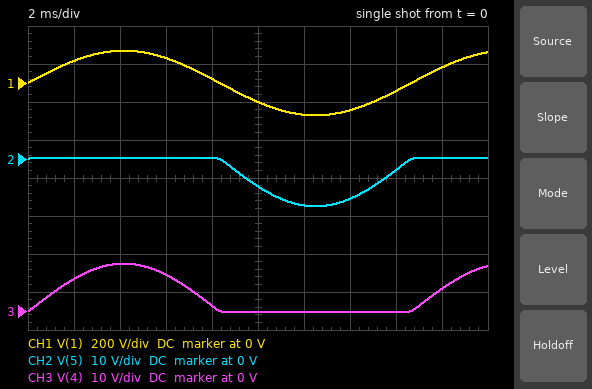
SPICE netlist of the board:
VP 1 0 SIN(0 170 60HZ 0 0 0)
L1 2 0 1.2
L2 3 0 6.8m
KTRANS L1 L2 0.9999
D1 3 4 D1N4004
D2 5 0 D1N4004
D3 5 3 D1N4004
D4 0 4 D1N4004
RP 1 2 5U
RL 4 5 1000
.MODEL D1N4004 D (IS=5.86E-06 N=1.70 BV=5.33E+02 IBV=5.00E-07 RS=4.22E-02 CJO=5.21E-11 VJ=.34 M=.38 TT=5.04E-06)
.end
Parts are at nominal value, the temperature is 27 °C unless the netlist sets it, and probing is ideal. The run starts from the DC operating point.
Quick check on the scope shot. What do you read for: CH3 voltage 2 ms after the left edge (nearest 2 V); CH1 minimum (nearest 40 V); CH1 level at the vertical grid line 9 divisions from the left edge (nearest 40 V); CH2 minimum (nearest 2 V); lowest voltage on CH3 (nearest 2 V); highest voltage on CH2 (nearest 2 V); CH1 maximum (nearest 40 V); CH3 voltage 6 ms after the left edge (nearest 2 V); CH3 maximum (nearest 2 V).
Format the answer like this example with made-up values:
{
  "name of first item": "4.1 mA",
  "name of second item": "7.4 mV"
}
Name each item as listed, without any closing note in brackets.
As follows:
{
  "CH3 voltage 2 ms after the left edge": "8 V",
  "CH1 minimum": "-160 V",
  "CH1 level at the vertical grid line 9 divisions from the left edge": "80 V",
  "CH2 minimum": "-12 V",
  "lowest voltage on CH3": "0 V",
  "highest voltage on CH2": "0 V",
  "CH1 maximum": "160 V",
  "CH3 voltage 6 ms after the left edge": "10 V",
  "CH3 maximum": "12 V"
}
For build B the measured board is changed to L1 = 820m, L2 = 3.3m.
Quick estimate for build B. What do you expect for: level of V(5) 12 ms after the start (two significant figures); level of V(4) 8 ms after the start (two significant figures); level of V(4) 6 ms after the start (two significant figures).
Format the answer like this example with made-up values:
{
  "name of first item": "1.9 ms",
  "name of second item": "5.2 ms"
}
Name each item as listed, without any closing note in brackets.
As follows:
{
  "level of V(5) 12 ms after the start": "-10 V",
  "level of V(4) 8 ms after the start": "1.1 V",
  "level of V(4) 6 ms after the start": "8.0 V"
}
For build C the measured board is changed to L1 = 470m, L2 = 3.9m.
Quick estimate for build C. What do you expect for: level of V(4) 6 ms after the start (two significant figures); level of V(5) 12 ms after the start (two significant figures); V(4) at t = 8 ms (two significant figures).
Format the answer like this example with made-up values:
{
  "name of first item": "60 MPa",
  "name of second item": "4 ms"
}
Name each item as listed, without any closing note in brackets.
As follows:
{
  "level of V(4) 6 ms after the start": "12 V",
  "level of V(5) 12 ms after the start": "-15 V",
  "V(4) at t = 8 ms": "1.7 V"
}
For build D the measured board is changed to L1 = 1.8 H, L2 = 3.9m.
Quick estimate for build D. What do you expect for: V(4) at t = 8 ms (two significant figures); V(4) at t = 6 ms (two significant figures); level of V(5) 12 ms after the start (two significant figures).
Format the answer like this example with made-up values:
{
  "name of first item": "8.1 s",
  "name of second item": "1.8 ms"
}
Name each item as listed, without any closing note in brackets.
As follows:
{
  "V(4) at t = 8 ms": "790 mV",
  "V(4) at t = 6 ms": "5.8 V",
  "level of V(5) 12 ms after the start": "-7.5 V"
}
